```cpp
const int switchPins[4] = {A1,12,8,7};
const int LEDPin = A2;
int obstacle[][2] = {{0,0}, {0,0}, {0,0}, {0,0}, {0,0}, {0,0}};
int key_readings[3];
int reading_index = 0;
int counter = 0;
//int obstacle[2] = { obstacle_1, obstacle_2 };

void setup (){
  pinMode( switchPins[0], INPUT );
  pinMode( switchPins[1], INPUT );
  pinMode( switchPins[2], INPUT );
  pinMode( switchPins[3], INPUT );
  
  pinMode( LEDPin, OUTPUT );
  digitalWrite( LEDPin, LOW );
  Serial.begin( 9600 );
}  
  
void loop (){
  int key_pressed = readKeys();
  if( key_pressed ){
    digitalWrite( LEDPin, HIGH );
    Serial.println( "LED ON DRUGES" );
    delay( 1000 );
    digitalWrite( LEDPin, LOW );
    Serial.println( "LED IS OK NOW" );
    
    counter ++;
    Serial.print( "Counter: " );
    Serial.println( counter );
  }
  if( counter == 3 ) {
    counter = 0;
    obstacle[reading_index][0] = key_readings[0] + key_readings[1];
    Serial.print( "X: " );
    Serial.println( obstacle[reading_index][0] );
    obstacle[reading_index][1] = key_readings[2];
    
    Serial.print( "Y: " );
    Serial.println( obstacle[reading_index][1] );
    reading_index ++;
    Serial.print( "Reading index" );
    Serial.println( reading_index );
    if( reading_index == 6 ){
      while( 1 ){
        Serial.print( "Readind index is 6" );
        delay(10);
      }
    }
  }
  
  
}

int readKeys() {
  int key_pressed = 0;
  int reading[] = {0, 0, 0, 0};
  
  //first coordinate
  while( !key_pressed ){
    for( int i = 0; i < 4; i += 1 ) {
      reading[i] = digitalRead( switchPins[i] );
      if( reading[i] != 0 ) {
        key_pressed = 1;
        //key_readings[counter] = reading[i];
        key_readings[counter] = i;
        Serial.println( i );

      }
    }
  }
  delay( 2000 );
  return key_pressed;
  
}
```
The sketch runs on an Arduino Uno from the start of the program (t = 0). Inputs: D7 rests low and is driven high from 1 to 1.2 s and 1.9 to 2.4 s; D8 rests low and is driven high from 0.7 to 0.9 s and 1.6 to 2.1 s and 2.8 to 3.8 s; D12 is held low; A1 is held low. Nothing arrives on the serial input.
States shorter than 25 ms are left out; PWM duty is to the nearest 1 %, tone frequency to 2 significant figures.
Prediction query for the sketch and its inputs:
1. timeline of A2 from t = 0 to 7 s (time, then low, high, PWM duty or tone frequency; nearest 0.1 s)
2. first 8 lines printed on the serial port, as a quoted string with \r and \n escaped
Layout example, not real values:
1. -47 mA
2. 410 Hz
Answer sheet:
1. 0 s low; 2.7 s high; 3.7 s low; 5.7 s high; 6.7 s low
2. "2\r\nLED ON DRUGES\r\nLED IS OK NOW\r\nCounter: 1\r\n2\r\nLED ON DRUGES\r\nLED IS OK NOW\r\nCounter: 2\r\n"
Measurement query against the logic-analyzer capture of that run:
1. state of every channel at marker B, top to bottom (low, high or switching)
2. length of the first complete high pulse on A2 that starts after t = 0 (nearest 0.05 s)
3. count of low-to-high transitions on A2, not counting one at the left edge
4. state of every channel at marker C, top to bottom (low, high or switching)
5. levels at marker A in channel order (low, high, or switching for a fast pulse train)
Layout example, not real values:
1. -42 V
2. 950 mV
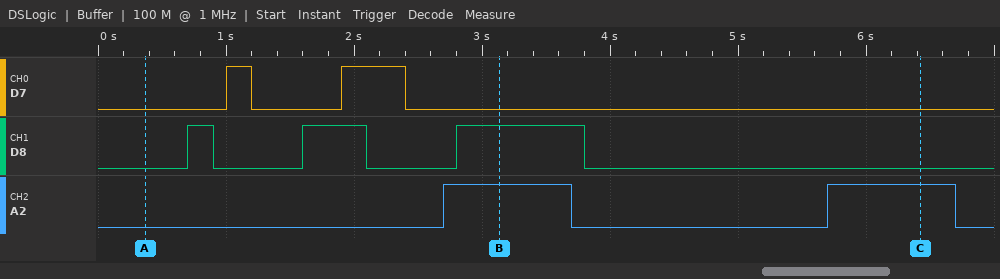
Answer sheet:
1. D7 low, D8 high, A2 high
2. 1.00 s
3. 2
4. D7 low, D8 low, A2 high
5. D7 low, D8 low, A2 low
